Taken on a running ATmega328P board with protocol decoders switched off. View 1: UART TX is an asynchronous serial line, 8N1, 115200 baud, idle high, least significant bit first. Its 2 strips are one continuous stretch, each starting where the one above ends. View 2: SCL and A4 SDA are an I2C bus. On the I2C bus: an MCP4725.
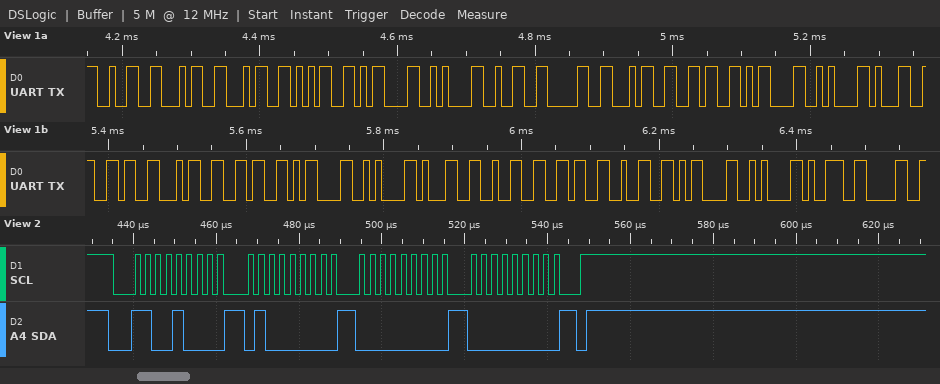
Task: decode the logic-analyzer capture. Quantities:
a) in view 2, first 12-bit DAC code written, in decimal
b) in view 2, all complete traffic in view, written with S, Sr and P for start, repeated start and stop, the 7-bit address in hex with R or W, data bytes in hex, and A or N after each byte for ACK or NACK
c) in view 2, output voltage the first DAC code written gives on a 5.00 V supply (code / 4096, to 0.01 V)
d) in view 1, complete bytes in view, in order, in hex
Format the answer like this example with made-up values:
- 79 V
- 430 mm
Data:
- 0
- S 64W A 40 A 00 A 00 A P
- 0.00 V
- 0x32 0x34 0x34 0x35 0x0D 0x0A 0x32 0x30 0x34 0x36 0x0D 0x0A 0x31 0x36 0x34 0x36 0x0D 0x0A 0x31 0x32 0x36 0x32 0x0D 0x0A 0x39 0x30
